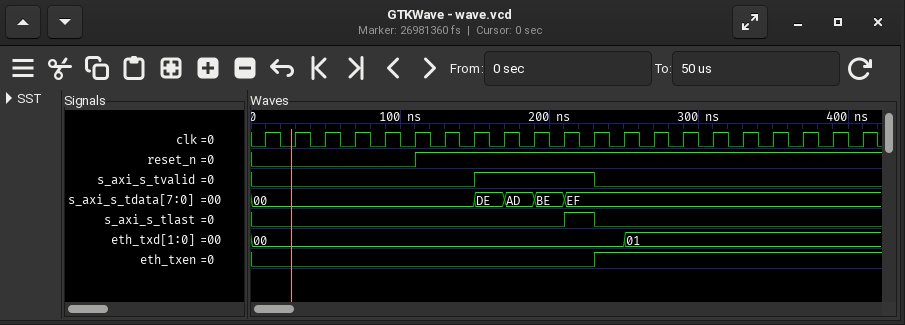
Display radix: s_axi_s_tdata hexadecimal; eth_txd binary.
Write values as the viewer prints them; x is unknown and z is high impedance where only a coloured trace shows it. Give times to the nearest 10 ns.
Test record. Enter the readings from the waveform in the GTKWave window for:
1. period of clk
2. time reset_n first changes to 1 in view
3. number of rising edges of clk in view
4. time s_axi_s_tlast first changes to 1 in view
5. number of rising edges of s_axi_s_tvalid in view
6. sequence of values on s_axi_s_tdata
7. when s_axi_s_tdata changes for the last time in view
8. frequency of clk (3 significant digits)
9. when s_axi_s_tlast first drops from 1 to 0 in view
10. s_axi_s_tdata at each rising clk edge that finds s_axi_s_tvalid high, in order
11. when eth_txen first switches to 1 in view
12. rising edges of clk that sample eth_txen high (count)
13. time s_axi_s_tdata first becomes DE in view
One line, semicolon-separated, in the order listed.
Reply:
20 ns; 110 ns; 21; 210 ns; 1; 00, DE, AD, BE, EF; 210 ns; 50.0 MHz; 230 ns; DE, AD, BE, EF; 230 ns; 9; 150 ns
